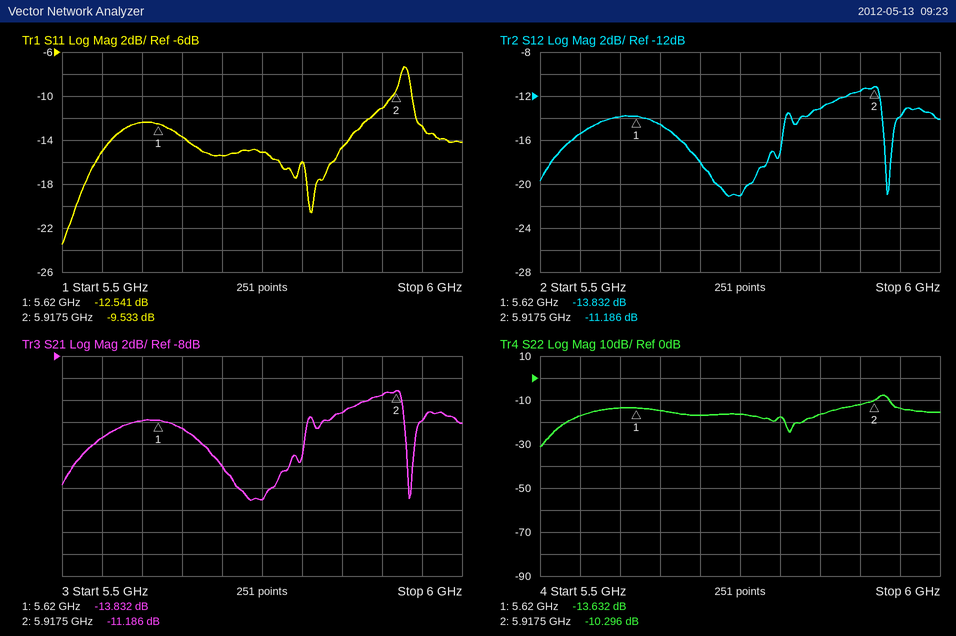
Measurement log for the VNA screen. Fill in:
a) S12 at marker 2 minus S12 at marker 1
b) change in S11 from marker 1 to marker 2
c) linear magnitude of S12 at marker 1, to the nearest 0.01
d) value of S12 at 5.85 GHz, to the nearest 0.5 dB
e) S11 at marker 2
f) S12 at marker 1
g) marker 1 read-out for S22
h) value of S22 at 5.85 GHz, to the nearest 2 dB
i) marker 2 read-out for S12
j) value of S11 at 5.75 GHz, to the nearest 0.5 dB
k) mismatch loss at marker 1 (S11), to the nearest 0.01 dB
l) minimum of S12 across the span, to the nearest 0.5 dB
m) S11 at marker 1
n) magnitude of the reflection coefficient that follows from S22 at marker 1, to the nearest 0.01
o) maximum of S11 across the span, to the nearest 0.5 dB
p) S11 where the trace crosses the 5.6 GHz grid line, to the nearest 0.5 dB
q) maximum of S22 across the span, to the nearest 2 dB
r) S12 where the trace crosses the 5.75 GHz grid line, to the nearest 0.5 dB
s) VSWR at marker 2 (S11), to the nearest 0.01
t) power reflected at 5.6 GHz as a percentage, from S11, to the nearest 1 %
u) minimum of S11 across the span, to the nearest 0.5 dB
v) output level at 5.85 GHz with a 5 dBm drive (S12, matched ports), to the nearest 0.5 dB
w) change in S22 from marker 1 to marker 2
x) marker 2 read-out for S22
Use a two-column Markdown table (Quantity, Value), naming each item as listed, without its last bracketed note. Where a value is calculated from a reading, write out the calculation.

| Quantity | Value |
|---|---|
| S12 at marker 2 minus S12 at marker 1 | -11.186 − (-13.832) = 2.646 dB |
| change in S11 from marker 1 to marker 2 | -9.533 − (-12.541) = 3.008 dB |
| linear magnitude of S12 at marker 1, to the nearest 0.01 | 10^(-13.832/20) ≈ 0.20 |
| value of S12 at 5.85 GHz, to the nearest 0.5 dB | -13.0 dB |
| S11 at marker 2 | -9.533 dB |
| S12 at marker 1 | -13.832 dB |
| marker 1 read-out for S22 | -13.632 dB |
| value of S22 at 5.85 GHz, to the nearest 2 dB | -16 dB |
| marker 2 read-out for S12 | -11.186 dB |
| value of S11 at 5.75 GHz, to the nearest 0.5 dB | -15.0 dB |
| mismatch loss at marker 1 (S11), to the nearest 0.01 dB | −10 log10(1 − 10^(-12.541/10)) ≈ 0.25 dB |
| minimum of S12 across the span, to the nearest 0.5 dB | -21.0 dB |
| S11 at marker 1 | -12.541 dB |
| magnitude of the reflection coefficient that follows from S22 at marker 1, to the nearest 0.01 | 10^(-13.632/20) ≈ 0.21 |
| maximum of S11 across the span, to the nearest 0.5 dB | -7.5 dB |
| S11 where the trace crosses the 5.6 GHz grid line, to the nearest 0.5 dB | -12.5 dB |
| maximum of S22 across the span, to the nearest 2 dB | -8 dB |
| S12 where the trace crosses the 5.75 GHz grid line, to the nearest 0.5 dB | -21.0 dB |
| VSWR at marker 2 (S11), to the nearest 0.01 | (1 + 0.3337)/(1 − 0.3337) ≈ 2.00 |
| power reflected at 5.6 GHz as a percentage, from S11, to the nearest 1 % | 10^(-12.5/10) ≈ 6 % |
| minimum of S11 across the span, to the nearest 0.5 dB | -23.5 dB |
| output level at 5.85 GHz with a 5 dBm drive (S12, matched ports), to the nearest 0.5 dB | 5 dBm + (-13.0 dB) = -8.0 dBm |
| change in S22 from marker 1 to marker 2 | -10.296 − (-13.632) = 3.336 dB |
| marker 2 read-out for S22 | -10.296 dB |
